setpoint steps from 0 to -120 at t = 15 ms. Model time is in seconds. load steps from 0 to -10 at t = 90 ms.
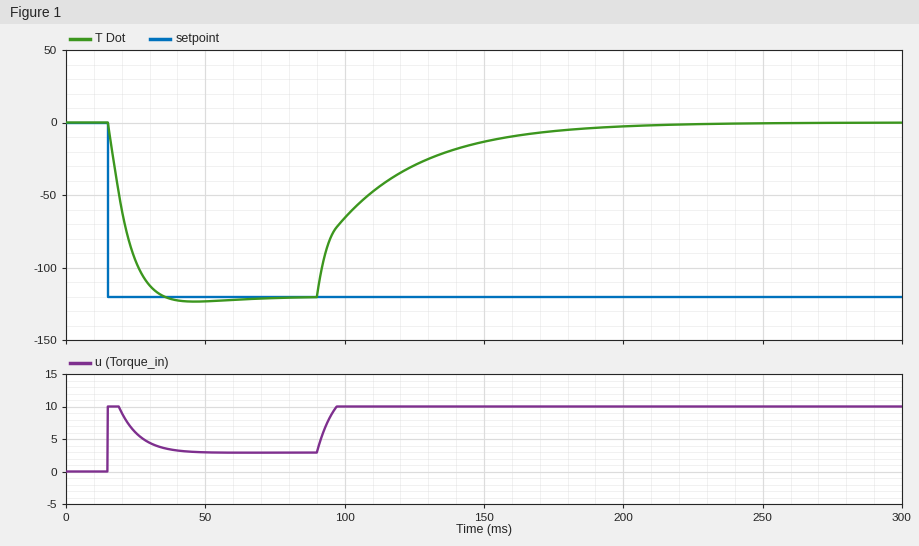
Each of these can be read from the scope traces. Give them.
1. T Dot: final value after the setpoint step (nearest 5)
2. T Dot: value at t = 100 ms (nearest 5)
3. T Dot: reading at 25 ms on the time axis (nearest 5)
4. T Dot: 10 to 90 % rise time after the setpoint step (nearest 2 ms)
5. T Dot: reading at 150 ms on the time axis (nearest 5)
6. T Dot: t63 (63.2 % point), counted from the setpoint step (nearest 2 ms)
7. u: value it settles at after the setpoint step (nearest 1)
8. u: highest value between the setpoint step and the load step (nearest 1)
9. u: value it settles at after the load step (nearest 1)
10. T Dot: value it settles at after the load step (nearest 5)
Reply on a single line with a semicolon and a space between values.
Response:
-120; -65; -95; 12 ms; -15; 6 ms; 3; 10; 10; 0
